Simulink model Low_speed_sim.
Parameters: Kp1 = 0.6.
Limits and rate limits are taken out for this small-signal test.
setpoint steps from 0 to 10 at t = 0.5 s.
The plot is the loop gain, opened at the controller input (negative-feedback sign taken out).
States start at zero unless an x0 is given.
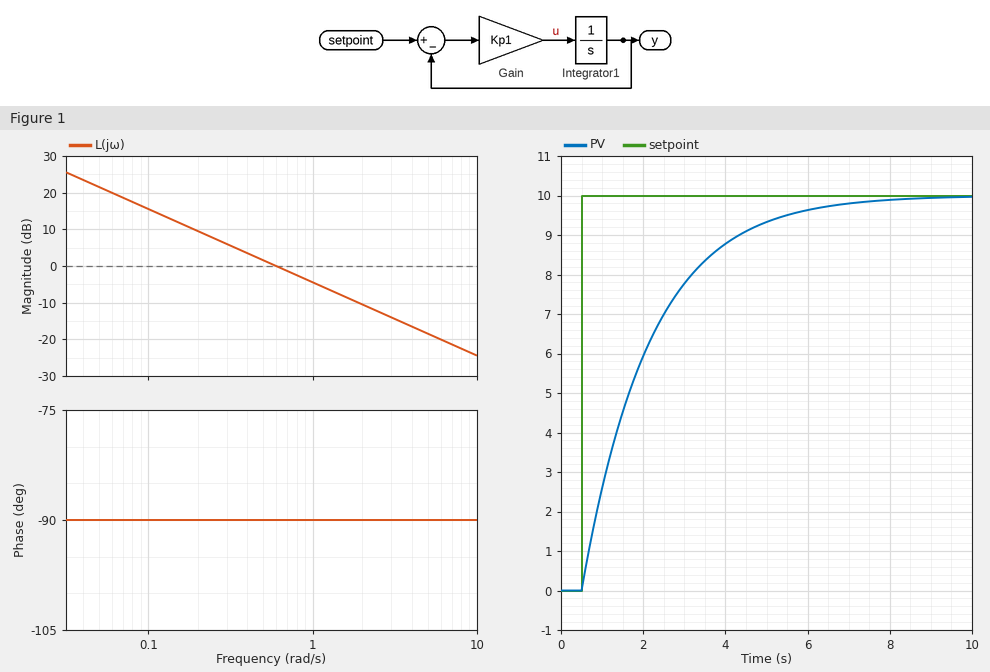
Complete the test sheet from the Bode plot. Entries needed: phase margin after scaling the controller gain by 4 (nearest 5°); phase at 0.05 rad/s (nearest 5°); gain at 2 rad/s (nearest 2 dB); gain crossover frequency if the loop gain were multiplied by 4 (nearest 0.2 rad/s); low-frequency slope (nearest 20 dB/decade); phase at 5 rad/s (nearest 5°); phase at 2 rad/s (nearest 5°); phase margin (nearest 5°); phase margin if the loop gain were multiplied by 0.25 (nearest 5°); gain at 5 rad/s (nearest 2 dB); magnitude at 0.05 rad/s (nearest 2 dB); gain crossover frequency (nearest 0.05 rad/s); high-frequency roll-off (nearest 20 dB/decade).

90°
-90°
-10 dB
2.4 rad/s
-20 dB/decade
-90°
-90°
90°
90°
-18 dB
22 dB
0.60 rad/s
-20 dB/decade
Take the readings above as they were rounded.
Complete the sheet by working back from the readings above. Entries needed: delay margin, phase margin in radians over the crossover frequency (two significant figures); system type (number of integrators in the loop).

2.6 s
1
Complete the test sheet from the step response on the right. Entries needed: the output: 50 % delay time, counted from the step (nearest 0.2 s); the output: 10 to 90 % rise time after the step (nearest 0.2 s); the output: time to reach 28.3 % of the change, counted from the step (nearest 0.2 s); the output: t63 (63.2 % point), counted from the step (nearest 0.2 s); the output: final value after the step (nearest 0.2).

1.2 s
3.6 s
0.6 s
1.6 s
10.0
